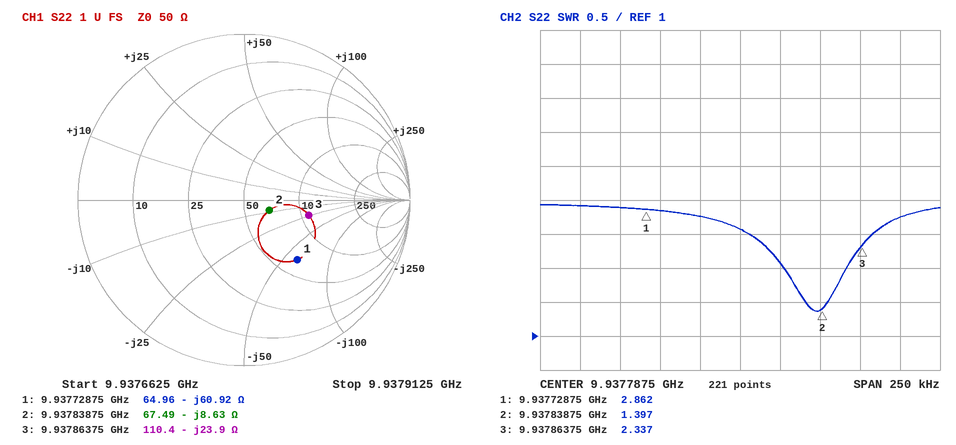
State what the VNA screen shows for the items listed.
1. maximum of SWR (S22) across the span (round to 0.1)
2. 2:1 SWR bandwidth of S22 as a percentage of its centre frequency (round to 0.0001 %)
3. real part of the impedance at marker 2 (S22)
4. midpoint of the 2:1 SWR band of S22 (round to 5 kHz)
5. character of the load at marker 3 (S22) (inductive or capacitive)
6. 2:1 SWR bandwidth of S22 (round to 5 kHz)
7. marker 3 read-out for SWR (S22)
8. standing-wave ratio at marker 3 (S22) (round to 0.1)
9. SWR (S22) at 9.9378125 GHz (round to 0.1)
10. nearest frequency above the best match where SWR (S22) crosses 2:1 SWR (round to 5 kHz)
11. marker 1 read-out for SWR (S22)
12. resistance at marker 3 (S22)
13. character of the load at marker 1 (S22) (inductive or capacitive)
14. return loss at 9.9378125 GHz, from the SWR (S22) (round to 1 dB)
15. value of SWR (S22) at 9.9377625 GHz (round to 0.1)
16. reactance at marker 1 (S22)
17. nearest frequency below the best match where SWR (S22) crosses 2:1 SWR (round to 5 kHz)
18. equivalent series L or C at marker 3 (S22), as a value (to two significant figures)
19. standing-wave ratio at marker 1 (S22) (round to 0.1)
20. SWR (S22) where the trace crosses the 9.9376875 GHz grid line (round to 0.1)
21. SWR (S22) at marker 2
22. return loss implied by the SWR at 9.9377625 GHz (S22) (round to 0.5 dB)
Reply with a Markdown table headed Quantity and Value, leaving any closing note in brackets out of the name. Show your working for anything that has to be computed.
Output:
| Quantity | Value |
|---|---|
| maximum of SWR (S22) across the span | 2.9 |
| 2:1 SWR bandwidth of S22 as a percentage of its centre frequency | 40 kHz / 9.93784 GHz ≈ 0.0004 % |
| real part of the impedance at marker 2 | 67.49 Ω |
| midpoint of the 2:1 SWR band of S22 | 9.937835 GHz |
| character of the load at marker 3 (S22) | capacitive |
| 2:1 SWR bandwidth of S22 | 9.937855 GHz − 9.937815 GHz = 40 kHz |
| marker 3 read-out for SWR | 2.337 |
| standing-wave ratio at marker 3 (S22) | 2.3 |
| SWR (S22) at 9.9378125 GHz | 2.1 |
| nearest frequency above the best match where SWR (S22) crosses 2:1 SWR | 9.937855 GHz |
| marker 1 read-out for SWR | 2.862 |
| resistance at marker 3 | 110.4 Ω |
| character of the load at marker 1 (S22) | capacitive |
| return loss at 9.9378125 GHz, from the SWR (S22) | −20 log10((2.1 − 1)/(2.1 + 1)) ≈ 9 dB |
| value of SWR (S22) at 9.9377625 GHz | 2.8 |
| reactance at marker 1 | -60.92 Ω |
| nearest frequency below the best match where SWR (S22) crosses 2:1 SWR | 9.937815 GHz |
| equivalent series L or C at marker 3 (S22), as a value | C = 1/(2π × 9.93786375 GHz × 23.9 Ω) ≈ 670 fF |
| standing-wave ratio at marker 1 (S22) | 2.9 |
| SWR (S22) where the trace crosses the 9.9376875 GHz grid line | 2.9 |
| SWR (S22) at marker 2 | 1.397 |
| return loss implied by the SWR at 9.9377625 GHz (S22) | −20 log10((2.8 − 1)/(2.8 + 1)) ≈ 6.5 dB |
